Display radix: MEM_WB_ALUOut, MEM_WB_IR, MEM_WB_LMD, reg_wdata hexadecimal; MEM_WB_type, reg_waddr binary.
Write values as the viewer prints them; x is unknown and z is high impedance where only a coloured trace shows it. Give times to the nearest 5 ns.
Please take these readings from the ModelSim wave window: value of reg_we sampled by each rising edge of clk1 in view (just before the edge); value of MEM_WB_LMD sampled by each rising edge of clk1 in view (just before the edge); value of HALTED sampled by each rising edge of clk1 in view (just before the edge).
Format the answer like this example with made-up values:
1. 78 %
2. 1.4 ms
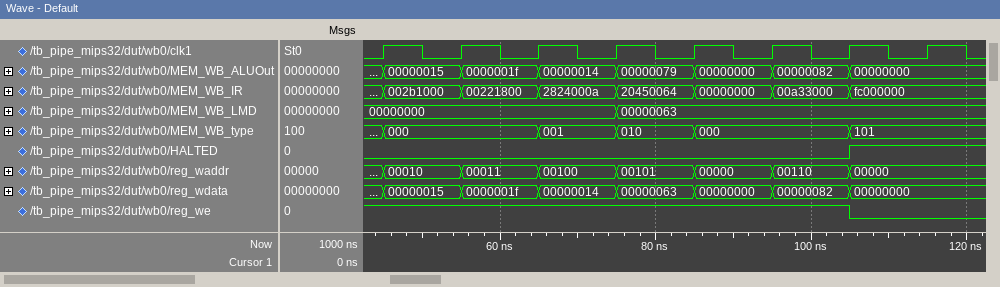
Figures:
1. 1 1 1 1 1 1 1 0
2. 00000000, 00000000, 00000000, 00000000, 00000063, 00000063, 00000063, 00000063
3. 0 0 0 0 0 0 0 1
